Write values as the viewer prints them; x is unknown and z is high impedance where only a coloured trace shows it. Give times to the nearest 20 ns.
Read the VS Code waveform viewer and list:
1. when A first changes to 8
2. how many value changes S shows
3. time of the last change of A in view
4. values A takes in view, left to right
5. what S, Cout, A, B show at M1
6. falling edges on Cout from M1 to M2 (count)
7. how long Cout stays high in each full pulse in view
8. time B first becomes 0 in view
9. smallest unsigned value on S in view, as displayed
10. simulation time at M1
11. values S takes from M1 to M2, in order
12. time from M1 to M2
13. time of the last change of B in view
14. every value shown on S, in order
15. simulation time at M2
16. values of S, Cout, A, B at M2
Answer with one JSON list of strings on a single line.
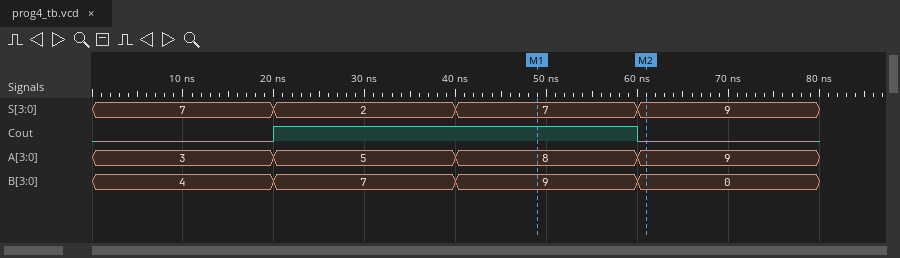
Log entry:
["40 ns", "3", "60 ns", "3, 5, 8, 9", "S=7, Cout=1, A=8, B=9", "1", "40 ns", "60 ns", "2", "40 ns", "7, 9", "20 ns", "60 ns", "7, 2, 7, 9", "60 ns", "S=9, Cout=0, A=9, B=0"]
